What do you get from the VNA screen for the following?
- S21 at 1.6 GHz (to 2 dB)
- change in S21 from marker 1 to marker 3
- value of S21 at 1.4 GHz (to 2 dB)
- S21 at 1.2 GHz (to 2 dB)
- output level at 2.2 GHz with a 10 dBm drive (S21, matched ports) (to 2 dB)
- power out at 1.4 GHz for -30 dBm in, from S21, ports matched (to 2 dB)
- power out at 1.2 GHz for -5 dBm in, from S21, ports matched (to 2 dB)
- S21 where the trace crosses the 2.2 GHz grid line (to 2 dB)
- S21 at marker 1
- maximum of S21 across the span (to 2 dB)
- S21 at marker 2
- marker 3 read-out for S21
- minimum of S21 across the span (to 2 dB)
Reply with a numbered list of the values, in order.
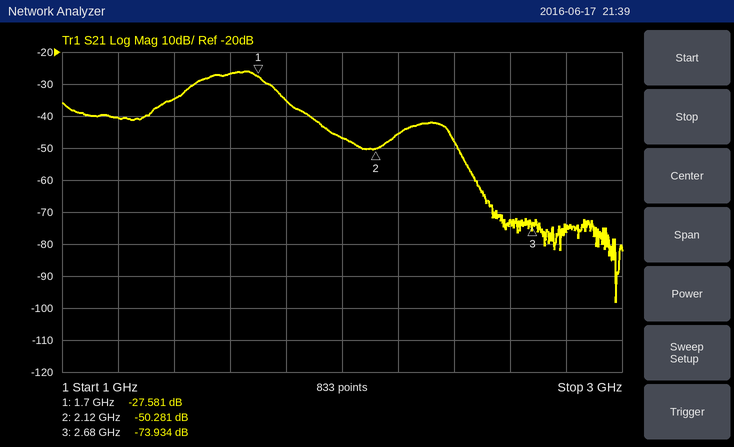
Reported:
1. -26 dB
2. -46.353 dB
3. -34 dB
4. -40 dB
5. -36 dBm
6. -64 dBm
7. -46 dBm
8. -46 dB
9. -27.581 dB
10. -26 dB
11. -50.281 dB
12. -73.934 dB
13. -98 dB
